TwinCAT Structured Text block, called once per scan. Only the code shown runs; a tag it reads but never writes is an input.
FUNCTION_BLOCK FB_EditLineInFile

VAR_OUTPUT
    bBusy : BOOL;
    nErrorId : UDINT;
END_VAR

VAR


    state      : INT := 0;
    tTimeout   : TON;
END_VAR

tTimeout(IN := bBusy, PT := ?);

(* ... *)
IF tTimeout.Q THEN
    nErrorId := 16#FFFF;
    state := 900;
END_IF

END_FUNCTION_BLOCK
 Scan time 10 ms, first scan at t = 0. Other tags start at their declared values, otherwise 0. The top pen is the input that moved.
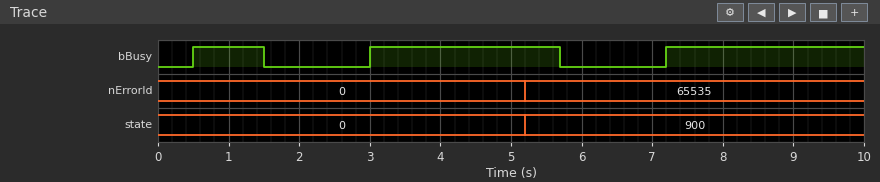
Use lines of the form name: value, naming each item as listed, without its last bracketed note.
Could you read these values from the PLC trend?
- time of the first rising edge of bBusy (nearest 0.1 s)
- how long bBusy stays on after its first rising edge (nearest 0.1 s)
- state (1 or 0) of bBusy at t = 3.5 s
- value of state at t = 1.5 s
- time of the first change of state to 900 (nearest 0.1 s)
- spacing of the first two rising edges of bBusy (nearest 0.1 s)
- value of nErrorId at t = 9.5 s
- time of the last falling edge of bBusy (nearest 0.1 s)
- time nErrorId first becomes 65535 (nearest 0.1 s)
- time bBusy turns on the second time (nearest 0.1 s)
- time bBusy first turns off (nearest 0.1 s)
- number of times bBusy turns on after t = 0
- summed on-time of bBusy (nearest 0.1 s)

time of the first rising edge of bBusy: 0.5 s
how long bBusy stays on after its first rising edge: 1.0 s
state (1 or 0) of bBusy at t = 3.5 s: 1
value of state at t = 1.5 s: 0
time of the first change of state to 900: 5.2 s
spacing of the first two rising edges of bBusy: 2.5 s
value of nErrorId at t = 9.5 s: 65535
time of the last falling edge of bBusy: 5.7 s
time nErrorId first becomes 65535: 5.2 s
time bBusy turns on the second time: 3.0 s
time bBusy first turns off: 1.5 s
number of times bBusy turns on after t = 0: 3
summed on-time of bBusy: 6.5 s
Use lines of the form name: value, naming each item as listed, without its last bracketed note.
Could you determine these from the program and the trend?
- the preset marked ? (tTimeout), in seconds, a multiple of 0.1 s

the preset marked ? (tTimeout), in seconds, a multiple of 0.1 s: 2.2 s
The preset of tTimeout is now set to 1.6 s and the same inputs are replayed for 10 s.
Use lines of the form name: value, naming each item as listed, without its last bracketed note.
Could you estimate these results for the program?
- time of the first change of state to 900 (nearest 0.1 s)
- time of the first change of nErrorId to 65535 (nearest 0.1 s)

time of the first change of state to 900: 4.6 s
time of the first change of nErrorId to 65535: 4.6 s
